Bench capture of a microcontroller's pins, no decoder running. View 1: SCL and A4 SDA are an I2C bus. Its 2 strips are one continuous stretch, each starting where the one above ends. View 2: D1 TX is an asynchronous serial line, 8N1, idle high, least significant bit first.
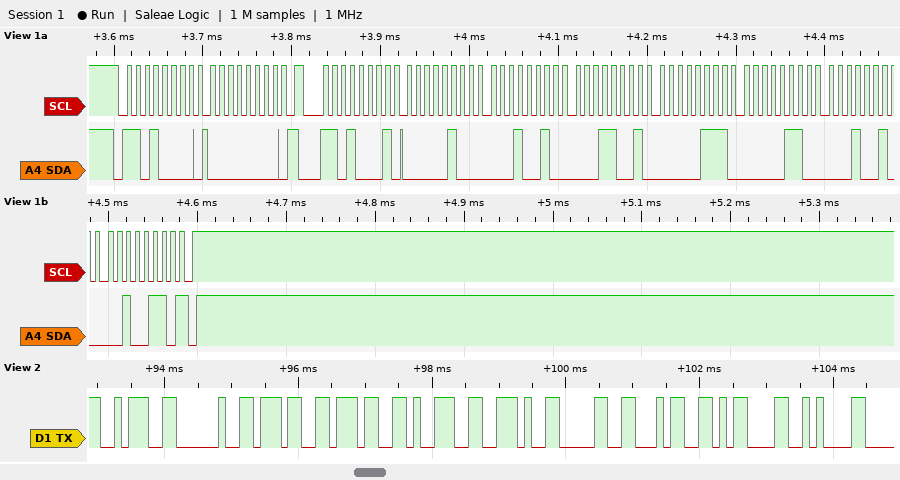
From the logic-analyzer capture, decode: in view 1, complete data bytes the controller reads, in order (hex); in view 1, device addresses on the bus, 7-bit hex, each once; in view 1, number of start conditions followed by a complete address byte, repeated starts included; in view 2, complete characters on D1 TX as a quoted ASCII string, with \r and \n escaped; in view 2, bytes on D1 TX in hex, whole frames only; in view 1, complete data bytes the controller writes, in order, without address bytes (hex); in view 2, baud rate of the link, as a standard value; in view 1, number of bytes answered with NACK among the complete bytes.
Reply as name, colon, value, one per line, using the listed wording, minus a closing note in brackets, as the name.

in view 1, complete data bytes the controller reads, in order: 04 12 19 07 06 12 26
in view 1, device addresses on the bus, 7-bit hex, each once: 0x68
in view 1, number of start conditions followed by a complete address byte, repeated starts included: 2
in view 2, complete characters on D1 TX as a quoted ASCII string, with \r and \n escaped: ": 779.04\r\n"
in view 2, bytes on D1 TX in hex, whole frames only: 3A 20 37 37 39 2E 30 34 0D 0A
in view 1, complete data bytes the controller writes, in order, without address bytes: 00
in view 2, baud rate of the link, as a standard value: 9600 baud
in view 1, number of bytes answered with NACK among the complete bytes: 1
